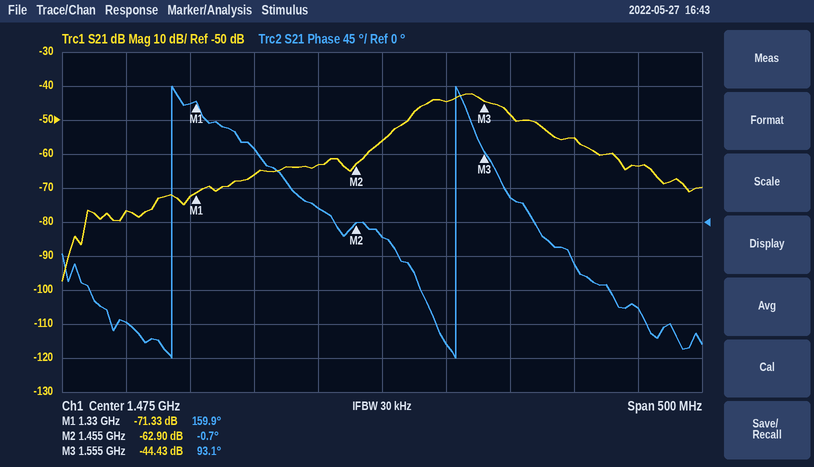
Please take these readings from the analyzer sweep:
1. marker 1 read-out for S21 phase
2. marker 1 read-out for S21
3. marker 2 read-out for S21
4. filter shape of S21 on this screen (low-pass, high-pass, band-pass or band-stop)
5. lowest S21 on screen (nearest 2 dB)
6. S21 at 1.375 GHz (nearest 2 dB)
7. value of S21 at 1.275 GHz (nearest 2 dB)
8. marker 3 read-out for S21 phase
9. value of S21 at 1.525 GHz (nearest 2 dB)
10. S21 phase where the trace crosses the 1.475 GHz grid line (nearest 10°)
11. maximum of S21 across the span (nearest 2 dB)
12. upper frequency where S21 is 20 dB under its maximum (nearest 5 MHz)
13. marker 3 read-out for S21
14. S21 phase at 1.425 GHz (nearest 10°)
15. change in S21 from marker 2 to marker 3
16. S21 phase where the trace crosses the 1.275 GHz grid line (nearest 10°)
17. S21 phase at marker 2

159.9°
-71.33 dB
-62.90 dB
band-pass
-98 dB
-66 dB
-76 dB
93.1°
-44 dB
-20°
-42 dB
1.660 GHz
-44.43 dB
20°
18.47 dB
-130°
-0.7°
